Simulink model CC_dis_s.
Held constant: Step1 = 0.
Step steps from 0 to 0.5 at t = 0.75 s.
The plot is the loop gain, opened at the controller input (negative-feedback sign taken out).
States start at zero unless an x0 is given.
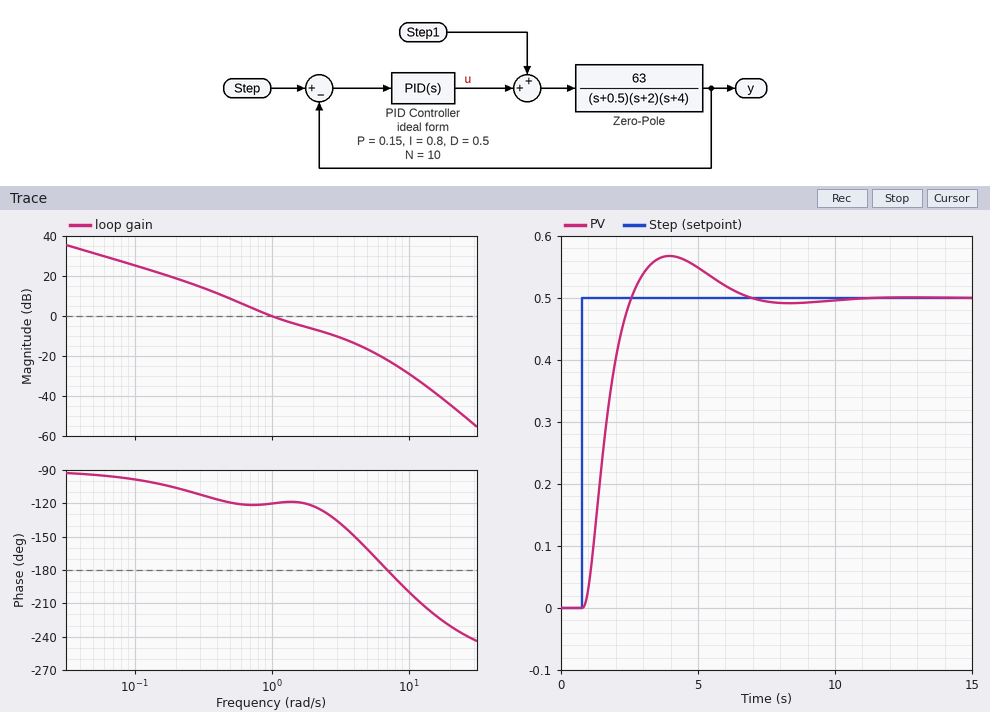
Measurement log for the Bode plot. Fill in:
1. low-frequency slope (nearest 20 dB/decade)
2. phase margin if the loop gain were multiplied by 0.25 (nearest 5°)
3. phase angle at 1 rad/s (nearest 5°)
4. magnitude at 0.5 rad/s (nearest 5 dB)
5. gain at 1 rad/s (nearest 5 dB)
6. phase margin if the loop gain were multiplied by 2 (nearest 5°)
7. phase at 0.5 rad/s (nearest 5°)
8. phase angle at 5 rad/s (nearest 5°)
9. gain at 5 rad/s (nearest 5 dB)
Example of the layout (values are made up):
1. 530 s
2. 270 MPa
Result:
1. -20 dB/decade
2. 65°
3. -120°
4. 10 dB
5. 0 dB
6. 60°
7. -120°
8. -160°
9. -15 dB
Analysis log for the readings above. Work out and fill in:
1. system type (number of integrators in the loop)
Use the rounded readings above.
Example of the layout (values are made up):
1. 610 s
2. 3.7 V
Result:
1. 1
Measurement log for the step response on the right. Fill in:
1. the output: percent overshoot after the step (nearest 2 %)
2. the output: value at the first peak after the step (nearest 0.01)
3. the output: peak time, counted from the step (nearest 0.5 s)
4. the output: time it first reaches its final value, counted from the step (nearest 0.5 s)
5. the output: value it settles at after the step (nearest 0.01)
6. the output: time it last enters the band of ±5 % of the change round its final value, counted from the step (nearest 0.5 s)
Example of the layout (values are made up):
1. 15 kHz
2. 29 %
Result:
1. 14 %
2. 0.57
3. 3.0 s
4. 2.0 s
5. 0.50
6. 5.0 s
